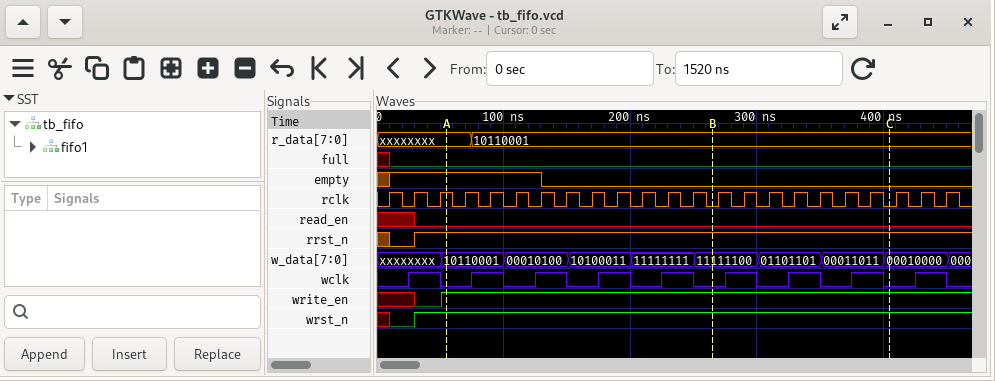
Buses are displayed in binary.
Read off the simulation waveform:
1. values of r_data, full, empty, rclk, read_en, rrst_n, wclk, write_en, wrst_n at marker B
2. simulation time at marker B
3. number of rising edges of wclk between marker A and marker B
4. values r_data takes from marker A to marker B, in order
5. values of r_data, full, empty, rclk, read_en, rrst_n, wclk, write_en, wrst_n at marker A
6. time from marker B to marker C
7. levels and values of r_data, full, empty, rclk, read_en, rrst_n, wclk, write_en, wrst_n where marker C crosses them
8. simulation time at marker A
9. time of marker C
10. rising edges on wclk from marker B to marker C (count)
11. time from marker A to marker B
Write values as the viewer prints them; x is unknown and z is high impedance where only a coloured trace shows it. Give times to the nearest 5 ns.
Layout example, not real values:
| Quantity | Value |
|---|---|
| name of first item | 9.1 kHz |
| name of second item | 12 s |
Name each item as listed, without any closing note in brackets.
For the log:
| Quantity | Value |
|---|---|
| values of r_data, full, empty, rclk, read_en, rrst_n, wclk, write_en, wrst_n at marker B | r_data=10110001, full=0, empty=0, rclk=0, read_en=0, rrst_n=1, wclk=0, write_en=1, wrst_n=1 |
| simulation time at marker B | 265 ns |
| number of rising edges of wclk between marker A and marker B | 4 |
| values r_data takes from marker A to marker B, in order | xxxxxxxx, 10110001 |
| values of r_data, full, empty, rclk, read_en, rrst_n, wclk, write_en, wrst_n at marker A | r_data=xxxxxxxx, full=0, empty=1, rclk=1, read_en=0, rrst_n=1, wclk=0, write_en=1, wrst_n=1 |
| time from marker B to marker C | 140 ns |
| levels and values of r_data, full, empty, rclk, read_en, rrst_n, wclk, write_en, wrst_n where marker C crosses them | r_data=10110001, full=0, empty=0, rclk=0, read_en=0, rrst_n=1, wclk=0, write_en=1, wrst_n=1 |
| simulation time at marker A | 55 ns |
| time of marker C | 405 ns |
| rising edges on wclk from marker B to marker C | 3 |
| time from marker A to marker B | 210 ns |
